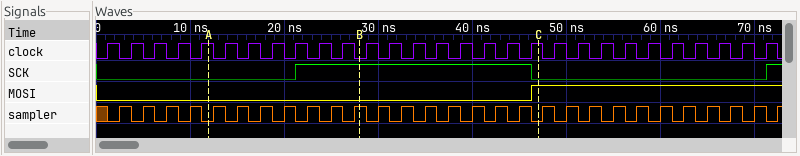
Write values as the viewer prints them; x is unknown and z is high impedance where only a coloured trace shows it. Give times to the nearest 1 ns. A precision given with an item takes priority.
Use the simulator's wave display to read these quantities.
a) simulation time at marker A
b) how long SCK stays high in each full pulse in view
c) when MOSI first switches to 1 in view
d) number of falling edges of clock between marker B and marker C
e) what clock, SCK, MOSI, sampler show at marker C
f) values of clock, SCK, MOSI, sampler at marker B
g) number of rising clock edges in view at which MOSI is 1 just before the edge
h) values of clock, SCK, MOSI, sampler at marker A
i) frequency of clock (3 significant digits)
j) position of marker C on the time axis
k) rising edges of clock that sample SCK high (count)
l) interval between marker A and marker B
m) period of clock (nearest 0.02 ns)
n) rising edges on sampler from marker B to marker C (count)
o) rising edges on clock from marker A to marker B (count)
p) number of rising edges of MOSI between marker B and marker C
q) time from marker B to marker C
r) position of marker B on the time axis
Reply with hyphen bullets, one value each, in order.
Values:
- 12 ns
- 25 ns
- 46 ns
- 7
- clock=1, SCK=0, MOSI=1, sampler=0
- clock=0, SCK=1, MOSI=0, sampler=1
- 10
- clock=1, SCK=0, MOSI=0, sampler=0
- 400 MHz
- 47 ns
- 10
- 16 ns
- 2.5 ns
- 7
- 6
- 1
- 19 ns
- 28 ns
